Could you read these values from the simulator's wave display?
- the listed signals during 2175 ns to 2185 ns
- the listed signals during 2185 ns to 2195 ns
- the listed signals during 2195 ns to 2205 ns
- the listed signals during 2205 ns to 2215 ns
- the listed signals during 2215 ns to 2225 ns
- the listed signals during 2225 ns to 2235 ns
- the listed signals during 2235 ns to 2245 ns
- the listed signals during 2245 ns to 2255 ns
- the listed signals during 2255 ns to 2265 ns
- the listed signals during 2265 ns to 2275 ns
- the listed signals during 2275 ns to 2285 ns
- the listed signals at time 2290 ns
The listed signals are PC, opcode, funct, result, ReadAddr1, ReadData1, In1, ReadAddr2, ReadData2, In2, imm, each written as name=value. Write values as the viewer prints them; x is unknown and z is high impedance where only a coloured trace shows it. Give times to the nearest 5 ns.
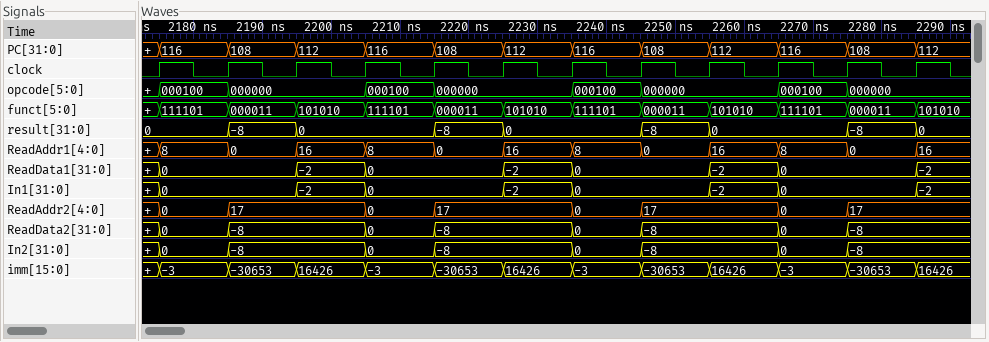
PC=116, opcode=000100, funct=111101, result=0, ReadAddr1=8, ReadData1=0, In1=0, ReadAddr2=0, ReadData2=0, In2=0, imm=-3
PC=108, opcode=000000, funct=000011, result=-8, ReadAddr1=0, ReadData1=0, In1=0, ReadAddr2=17, ReadData2=-8, In2=-8, imm=-30653
PC=112, opcode=000000, funct=101010, result=0, ReadAddr1=16, ReadData1=-2, In1=-2, ReadAddr2=17, ReadData2=-8, In2=-8, imm=16426
PC=116, opcode=000100, funct=111101, result=0, ReadAddr1=8, ReadData1=0, In1=0, ReadAddr2=0, ReadData2=0, In2=0, imm=-3
PC=108, opcode=000000, funct=000011, result=-8, ReadAddr1=0, ReadData1=0, In1=0, ReadAddr2=17, ReadData2=-8, In2=-8, imm=-30653
PC=112, opcode=000000, funct=101010, result=0, ReadAddr1=16, ReadData1=-2, In1=-2, ReadAddr2=17, ReadData2=-8, In2=-8, imm=16426
PC=116, opcode=000100, funct=111101, result=0, ReadAddr1=8, ReadData1=0, In1=0, ReadAddr2=0, ReadData2=0, In2=0, imm=-3
PC=108, opcode=000000, funct=000011, result=-8, ReadAddr1=0, ReadData1=0, In1=0, ReadAddr2=17, ReadData2=-8, In2=-8, imm=-30653
PC=112, opcode=000000, funct=101010, result=0, ReadAddr1=16, ReadData1=-2, In1=-2, ReadAddr2=17, ReadData2=-8, In2=-8, imm=16426
PC=116, opcode=000100, funct=111101, result=0, ReadAddr1=8, ReadData1=0, In1=0, ReadAddr2=0, ReadData2=0, In2=0, imm=-3
PC=108, opcode=000000, funct=000011, result=-8, ReadAddr1=0, ReadData1=0, In1=0, ReadAddr2=17, ReadData2=-8, In2=-8, imm=-30653
PC=112, opcode=000000, funct=101010, result=0, ReadAddr1=16, ReadData1=-2, In1=-2, ReadAddr2=17, ReadData2=-8, In2=-8, imm=16426
